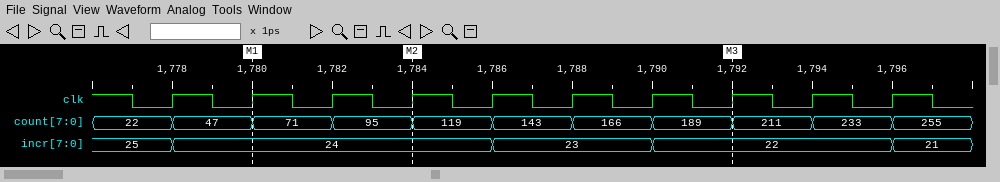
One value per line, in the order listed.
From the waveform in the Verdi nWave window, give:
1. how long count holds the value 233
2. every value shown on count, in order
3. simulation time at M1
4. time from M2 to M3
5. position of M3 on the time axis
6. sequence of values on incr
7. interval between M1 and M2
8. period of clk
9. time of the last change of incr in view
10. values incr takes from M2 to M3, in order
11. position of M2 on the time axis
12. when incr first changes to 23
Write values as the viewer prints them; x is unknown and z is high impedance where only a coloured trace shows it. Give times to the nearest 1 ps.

2 ps
22, 47, 71, 95, 119, 143, 166, 189, 211, 233, 255
1780 ps
8 ps
1792 ps
25, 24, 23, 22, 21
4 ps
2 ps
1796 ps
24, 23, 22
1784 ps
1786 ps
